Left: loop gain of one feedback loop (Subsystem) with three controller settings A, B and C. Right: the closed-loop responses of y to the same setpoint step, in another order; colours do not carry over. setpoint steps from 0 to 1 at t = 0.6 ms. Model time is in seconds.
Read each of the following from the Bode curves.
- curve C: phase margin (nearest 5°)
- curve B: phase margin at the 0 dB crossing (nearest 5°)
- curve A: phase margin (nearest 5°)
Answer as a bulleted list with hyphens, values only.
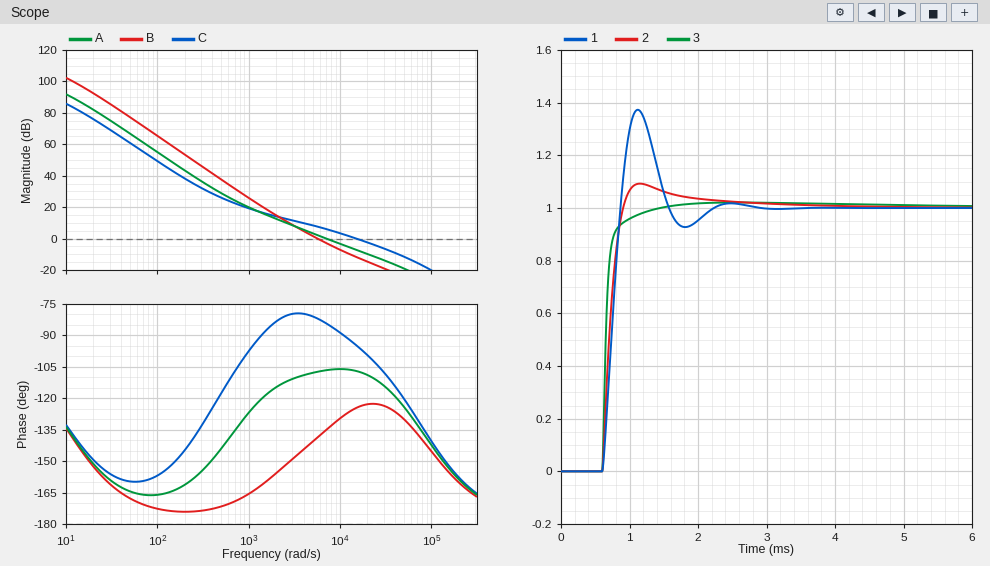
- 85°
- 40°
- 75°
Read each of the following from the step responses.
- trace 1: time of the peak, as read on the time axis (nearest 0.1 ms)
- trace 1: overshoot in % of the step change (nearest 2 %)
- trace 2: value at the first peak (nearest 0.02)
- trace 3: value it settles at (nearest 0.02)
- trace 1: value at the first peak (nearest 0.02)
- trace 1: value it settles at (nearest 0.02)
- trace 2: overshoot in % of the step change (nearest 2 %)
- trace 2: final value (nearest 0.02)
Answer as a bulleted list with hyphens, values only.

- 1.1 ms
- 38 %
- 1.10
- 1.00
- 1.38
- 1.00
- 10 %
- 1.00
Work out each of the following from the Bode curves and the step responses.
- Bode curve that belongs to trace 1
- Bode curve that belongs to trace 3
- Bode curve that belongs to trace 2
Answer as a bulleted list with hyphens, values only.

- B
- C
- A
